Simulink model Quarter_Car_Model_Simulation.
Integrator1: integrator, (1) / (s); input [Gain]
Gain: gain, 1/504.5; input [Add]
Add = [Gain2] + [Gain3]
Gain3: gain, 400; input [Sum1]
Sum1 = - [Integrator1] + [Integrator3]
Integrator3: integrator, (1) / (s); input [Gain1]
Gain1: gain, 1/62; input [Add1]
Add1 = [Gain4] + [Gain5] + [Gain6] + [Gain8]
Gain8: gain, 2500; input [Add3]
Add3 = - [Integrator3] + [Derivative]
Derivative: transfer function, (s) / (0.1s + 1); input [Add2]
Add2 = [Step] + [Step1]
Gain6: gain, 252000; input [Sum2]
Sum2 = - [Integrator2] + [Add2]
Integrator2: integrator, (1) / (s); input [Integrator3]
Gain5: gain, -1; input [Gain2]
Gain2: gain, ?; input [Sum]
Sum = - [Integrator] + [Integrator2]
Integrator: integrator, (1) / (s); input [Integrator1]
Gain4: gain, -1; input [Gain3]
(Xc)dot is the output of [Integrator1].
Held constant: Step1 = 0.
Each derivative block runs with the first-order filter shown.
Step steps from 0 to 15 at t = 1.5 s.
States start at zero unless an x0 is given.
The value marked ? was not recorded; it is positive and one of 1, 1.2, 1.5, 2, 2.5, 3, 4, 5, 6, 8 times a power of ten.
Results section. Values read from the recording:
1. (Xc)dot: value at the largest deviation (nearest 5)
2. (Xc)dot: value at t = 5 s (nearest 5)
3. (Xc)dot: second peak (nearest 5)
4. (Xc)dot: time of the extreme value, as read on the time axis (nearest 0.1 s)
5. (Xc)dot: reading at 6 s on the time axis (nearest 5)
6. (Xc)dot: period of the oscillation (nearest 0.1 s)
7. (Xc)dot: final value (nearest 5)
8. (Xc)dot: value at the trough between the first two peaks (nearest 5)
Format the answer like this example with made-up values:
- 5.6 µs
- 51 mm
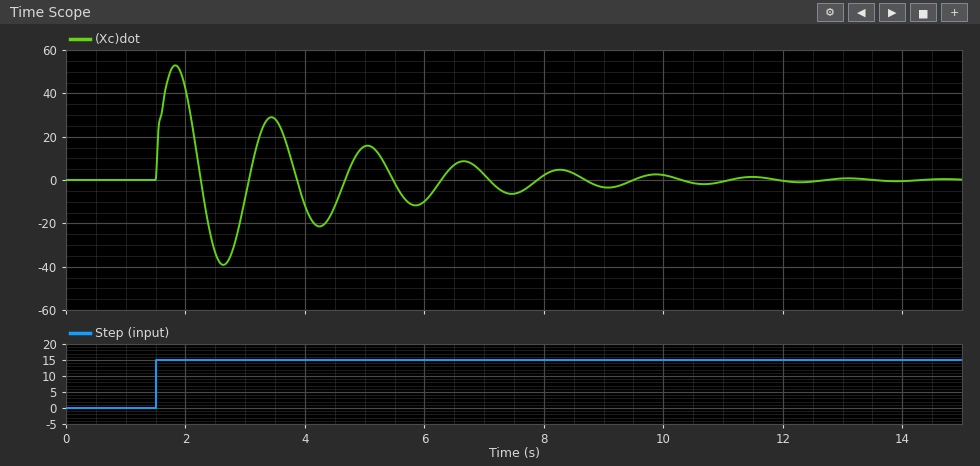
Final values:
- 55
- 15
- 30
- 1.8 s
- -10
- 1.6 s
- 0
- -40
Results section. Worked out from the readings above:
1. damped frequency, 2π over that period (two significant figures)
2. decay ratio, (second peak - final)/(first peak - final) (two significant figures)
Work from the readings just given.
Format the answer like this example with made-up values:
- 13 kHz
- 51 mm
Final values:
- 3.9 rad/s
- 0.55
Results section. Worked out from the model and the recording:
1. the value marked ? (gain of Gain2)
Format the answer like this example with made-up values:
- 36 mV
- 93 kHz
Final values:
- 8000
